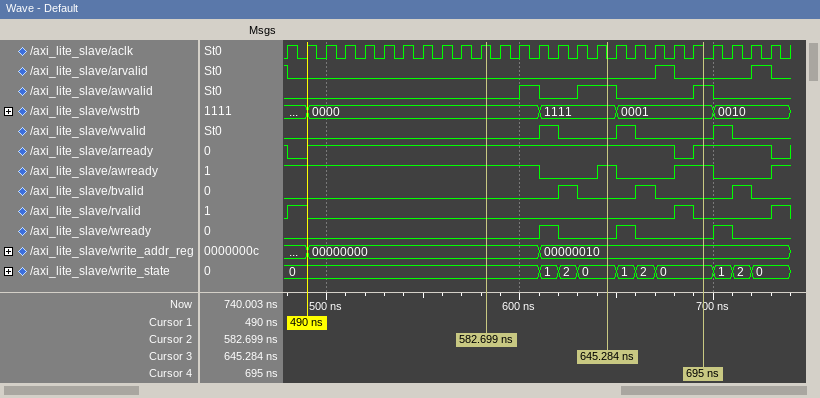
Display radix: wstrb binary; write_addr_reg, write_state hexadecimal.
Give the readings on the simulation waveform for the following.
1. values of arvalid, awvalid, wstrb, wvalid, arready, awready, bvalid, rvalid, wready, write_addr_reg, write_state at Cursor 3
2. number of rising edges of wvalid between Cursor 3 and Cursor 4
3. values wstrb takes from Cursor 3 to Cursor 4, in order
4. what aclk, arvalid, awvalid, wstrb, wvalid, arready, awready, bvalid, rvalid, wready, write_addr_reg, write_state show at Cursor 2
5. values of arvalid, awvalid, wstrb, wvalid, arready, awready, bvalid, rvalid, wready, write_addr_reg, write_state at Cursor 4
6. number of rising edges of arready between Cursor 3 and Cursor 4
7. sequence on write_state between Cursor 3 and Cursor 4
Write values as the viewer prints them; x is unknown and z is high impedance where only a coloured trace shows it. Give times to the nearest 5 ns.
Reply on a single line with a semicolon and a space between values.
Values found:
arvalid=0, awvalid=1, wstrb=1111, wvalid=0, arready=1, awready=1, bvalid=0, rvalid=0, wready=0, write_addr_reg=00000010, write_state=0; 1; 1111, 0001; aclk=1, arvalid=0, awvalid=0, wstrb=0000, wvalid=0, arready=1, awready=1, bvalid=0, rvalid=0, wready=0, write_addr_reg=00000000, write_state=0; arvalid=0, awvalid=1, wstrb=0001, wvalid=0, arready=1, awready=1, bvalid=0, rvalid=0, wready=0, write_addr_reg=00000010, write_state=0; 1; 0, 1, 2, 0
